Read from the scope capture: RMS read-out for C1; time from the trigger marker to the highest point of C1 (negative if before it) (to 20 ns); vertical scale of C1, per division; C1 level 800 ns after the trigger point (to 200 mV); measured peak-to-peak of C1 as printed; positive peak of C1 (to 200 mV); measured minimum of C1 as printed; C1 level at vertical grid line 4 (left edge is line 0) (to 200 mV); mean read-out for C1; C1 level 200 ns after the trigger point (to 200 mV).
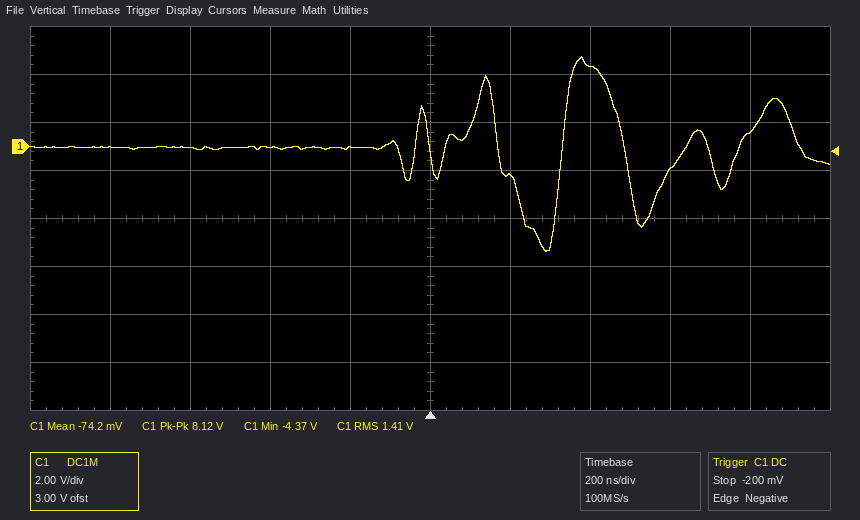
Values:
1.41 V
+380 ns
2 V
600 mV
8.12 V
3.8 V
-4.37 V
0.0 V
-74.2 mV
-1.2 V
